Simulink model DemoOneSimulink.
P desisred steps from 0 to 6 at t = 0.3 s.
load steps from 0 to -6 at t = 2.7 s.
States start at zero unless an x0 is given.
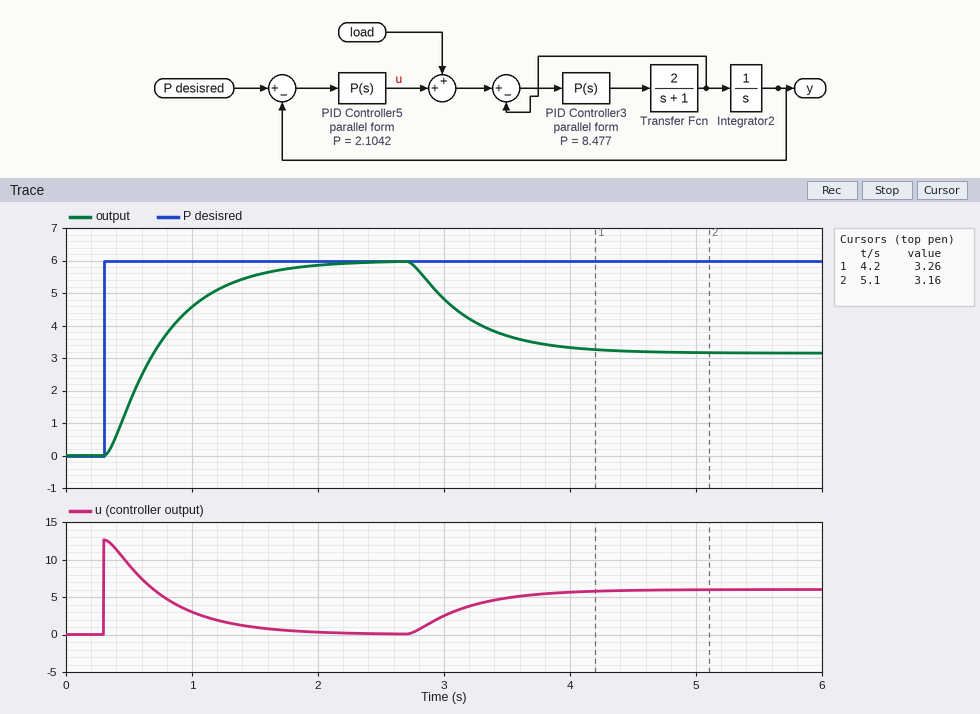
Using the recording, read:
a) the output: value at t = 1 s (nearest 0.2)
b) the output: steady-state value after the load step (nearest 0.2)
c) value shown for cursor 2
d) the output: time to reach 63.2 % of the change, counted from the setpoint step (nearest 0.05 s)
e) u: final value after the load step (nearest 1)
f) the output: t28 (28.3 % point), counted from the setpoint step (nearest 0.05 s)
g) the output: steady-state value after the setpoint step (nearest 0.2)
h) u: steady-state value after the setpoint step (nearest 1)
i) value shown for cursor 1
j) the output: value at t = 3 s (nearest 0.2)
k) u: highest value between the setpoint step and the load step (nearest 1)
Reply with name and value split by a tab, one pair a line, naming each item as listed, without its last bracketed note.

the output: value at t = 1 s	4.6
the output: steady-state value after the load step	3.2
value shown for cursor 2	3.16
the output: time to reach 63.2 % of the change, counted from the setpoint step	0.50 s
u: final value after the load step	6
the output: t28 (28.3 % point), counted from the setpoint step	0.20 s
the output: steady-state value after the setpoint step	6.0
u: steady-state value after the setpoint step	0
value shown for cursor 1	3.26
the output: value at t = 3 s	4.8
u: highest value between the setpoint step and the load step	13
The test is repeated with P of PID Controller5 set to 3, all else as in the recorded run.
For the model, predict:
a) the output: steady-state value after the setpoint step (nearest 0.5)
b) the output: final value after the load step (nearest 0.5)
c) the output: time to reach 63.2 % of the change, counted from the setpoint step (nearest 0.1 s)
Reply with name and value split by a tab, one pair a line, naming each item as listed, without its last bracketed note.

the output: steady-state value after the setpoint step	6.0
the output: final value after the load step	4.0
the output: time to reach 63.2 % of the change, counted from the setpoint step	0.4 s
